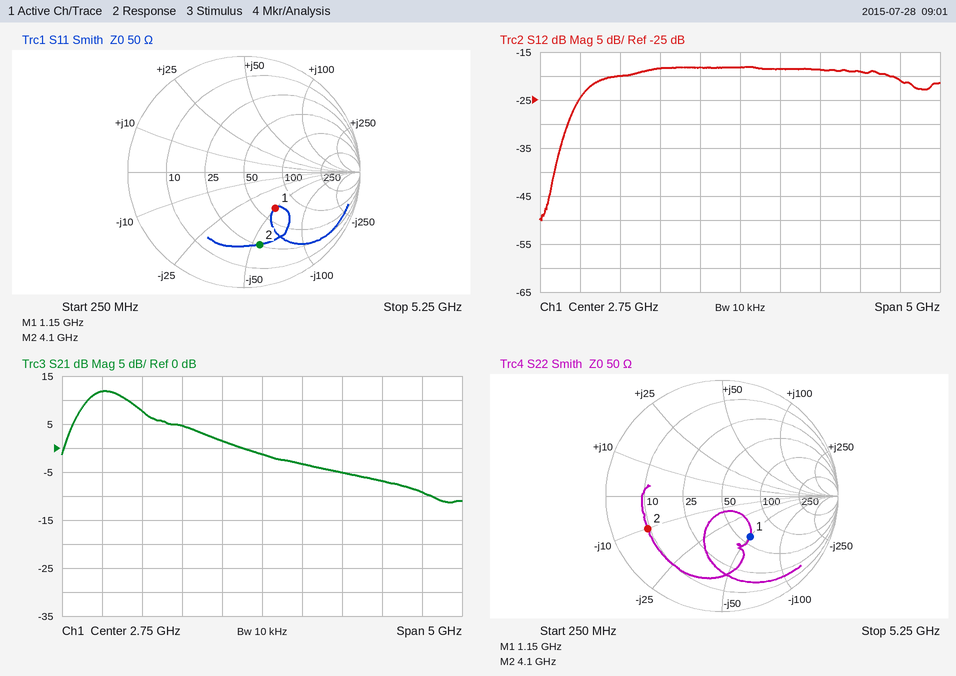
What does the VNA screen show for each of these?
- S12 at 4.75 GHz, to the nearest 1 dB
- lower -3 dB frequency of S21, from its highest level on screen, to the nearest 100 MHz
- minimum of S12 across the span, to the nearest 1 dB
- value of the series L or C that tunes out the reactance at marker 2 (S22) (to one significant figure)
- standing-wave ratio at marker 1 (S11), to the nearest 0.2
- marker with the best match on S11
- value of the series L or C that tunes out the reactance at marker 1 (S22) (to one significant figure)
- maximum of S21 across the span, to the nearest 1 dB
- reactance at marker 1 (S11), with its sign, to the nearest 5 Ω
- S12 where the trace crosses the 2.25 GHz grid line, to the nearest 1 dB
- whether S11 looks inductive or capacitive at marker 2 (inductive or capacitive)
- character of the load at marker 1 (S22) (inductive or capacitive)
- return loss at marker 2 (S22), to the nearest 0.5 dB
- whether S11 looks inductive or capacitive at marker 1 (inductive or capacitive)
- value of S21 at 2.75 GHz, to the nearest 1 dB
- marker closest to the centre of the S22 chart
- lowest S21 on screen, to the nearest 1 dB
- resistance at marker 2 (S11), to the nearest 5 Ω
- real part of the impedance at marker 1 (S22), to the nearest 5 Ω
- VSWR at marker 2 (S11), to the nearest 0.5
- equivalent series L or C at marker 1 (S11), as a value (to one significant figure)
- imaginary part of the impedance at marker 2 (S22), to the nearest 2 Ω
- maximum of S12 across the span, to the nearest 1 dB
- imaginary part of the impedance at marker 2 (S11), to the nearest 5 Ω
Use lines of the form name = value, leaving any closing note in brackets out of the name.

S12 at 4.75 GHz, to the nearest 1 dB = -21 dB
lower -3 dB frequency of S21, from its highest level on screen, to the nearest 100 MHz = 500 MHz
minimum of S12 across the span, to the nearest 1 dB = -50 dB
value of the series L or C that tunes out the reactance at marker 2 (S22) = 400 pH
standing-wave ratio at marker 1 (S11), to the nearest 0.2 = 2.4
marker with the best match on S11 = marker 1
value of the series L or C that tunes out the reactance at marker 1 (S22) = 7 nH
maximum of S21 across the span, to the nearest 1 dB = 12 dB
reactance at marker 1 (S11), with its sign, to the nearest 5 Ω = -50 Ω
S12 where the trace crosses the 2.25 GHz grid line, to the nearest 1 dB = -18 dB
whether S11 looks inductive or capacitive at marker 2 = capacitive
character of the load at marker 1 (S22) = capacitive
return loss at marker 2 (S22), to the nearest 0.5 dB = 3.0 dB
whether S11 looks inductive or capacitive at marker 1 = capacitive
value of S21 at 2.75 GHz, to the nearest 1 dB = -1 dB
marker closest to the centre of the S22 chart = marker 1
lowest S21 on screen, to the nearest 1 dB = -11 dB
resistance at marker 2 (S11), to the nearest 5 Ω = 25 Ω
real part of the impedance at marker 1 (S22), to the nearest 5 Ω = 60 Ω
VSWR at marker 2 (S11), to the nearest 0.5 = 4.5
equivalent series L or C at marker 1 (S11), as a value = 3 pF
imaginary part of the impedance at marker 2 (S22), to the nearest 2 Ω = -10 Ω
maximum of S12 across the span, to the nearest 1 dB = -18 dB
imaginary part of the impedance at marker 2 (S11), to the nearest 5 Ω = -55 Ω
